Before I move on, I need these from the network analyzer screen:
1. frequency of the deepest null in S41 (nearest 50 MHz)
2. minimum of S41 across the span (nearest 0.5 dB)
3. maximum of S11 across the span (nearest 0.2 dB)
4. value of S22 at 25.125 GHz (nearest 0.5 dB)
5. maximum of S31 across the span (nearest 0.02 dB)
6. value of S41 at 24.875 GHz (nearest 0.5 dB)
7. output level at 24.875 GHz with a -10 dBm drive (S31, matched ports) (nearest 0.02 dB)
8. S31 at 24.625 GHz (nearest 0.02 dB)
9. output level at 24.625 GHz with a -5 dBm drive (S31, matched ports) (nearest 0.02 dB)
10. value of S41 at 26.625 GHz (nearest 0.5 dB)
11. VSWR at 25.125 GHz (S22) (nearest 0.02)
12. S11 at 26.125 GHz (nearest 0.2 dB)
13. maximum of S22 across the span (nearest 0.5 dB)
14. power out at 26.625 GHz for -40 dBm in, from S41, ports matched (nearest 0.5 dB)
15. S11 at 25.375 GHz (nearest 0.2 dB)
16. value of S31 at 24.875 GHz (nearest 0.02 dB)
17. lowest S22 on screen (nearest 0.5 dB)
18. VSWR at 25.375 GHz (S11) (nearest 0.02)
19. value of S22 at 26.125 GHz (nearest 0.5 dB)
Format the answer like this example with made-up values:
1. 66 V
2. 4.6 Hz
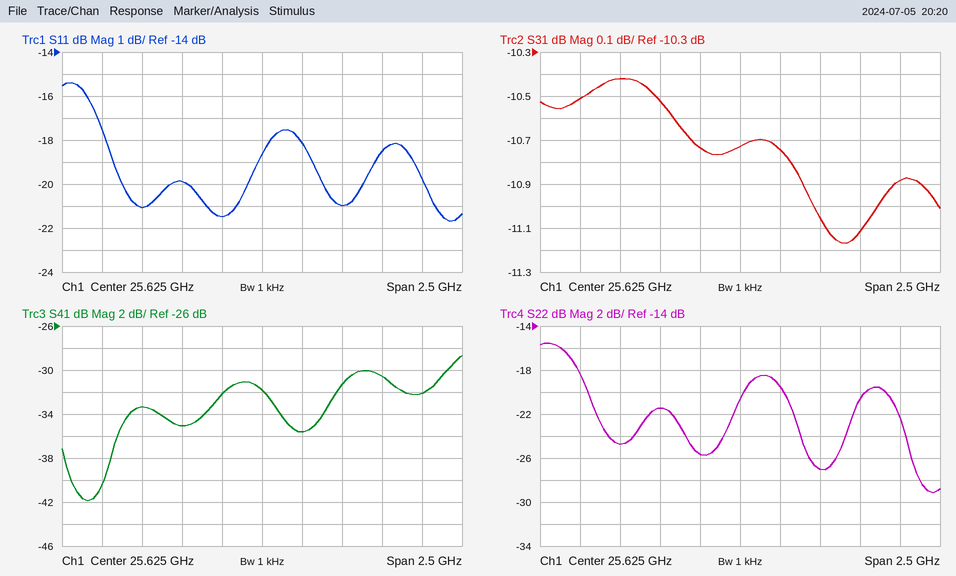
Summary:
1. 24.55 GHz
2. -42.0 dB
3. -15.4 dB
4. -21.5 dB
5. -10.42 dB
6. -33.5 dB
7. -20.42 dBm
8. -10.52 dB
9. -15.52 dBm
10. -32.0 dB
11. 1.18
12. -21.0 dB
13. -15.5 dB
14. -72.0 dBm
15. -21.4 dB
16. -10.42 dB
17. -29.0 dB
18. 1.18
19. -27.0 dB
